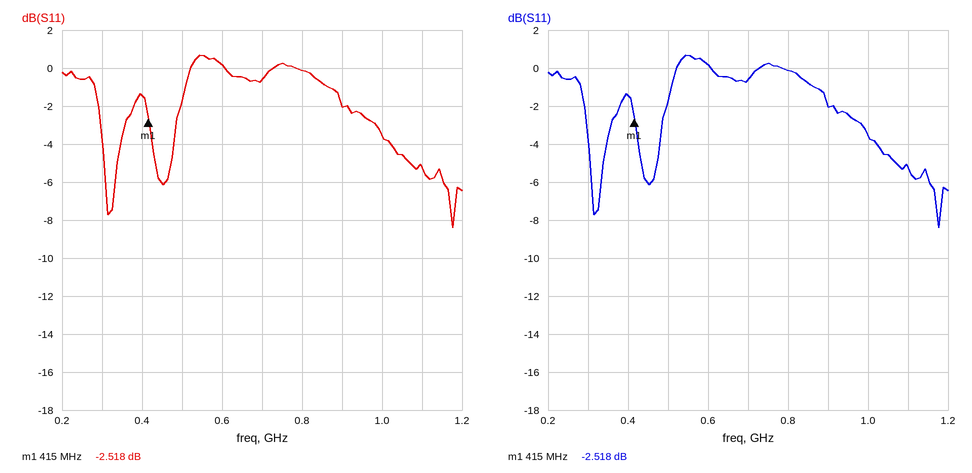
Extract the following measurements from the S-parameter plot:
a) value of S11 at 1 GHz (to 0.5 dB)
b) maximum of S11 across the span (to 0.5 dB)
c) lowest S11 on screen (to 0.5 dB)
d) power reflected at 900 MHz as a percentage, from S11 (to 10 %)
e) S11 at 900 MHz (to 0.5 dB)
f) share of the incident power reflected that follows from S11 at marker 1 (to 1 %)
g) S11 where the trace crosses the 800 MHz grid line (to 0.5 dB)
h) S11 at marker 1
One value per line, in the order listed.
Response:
-3.5 dB
0.5 dB
-8.5 dB
60 %
-2.0 dB
56 %
0.0 dB
-2.518 dB
